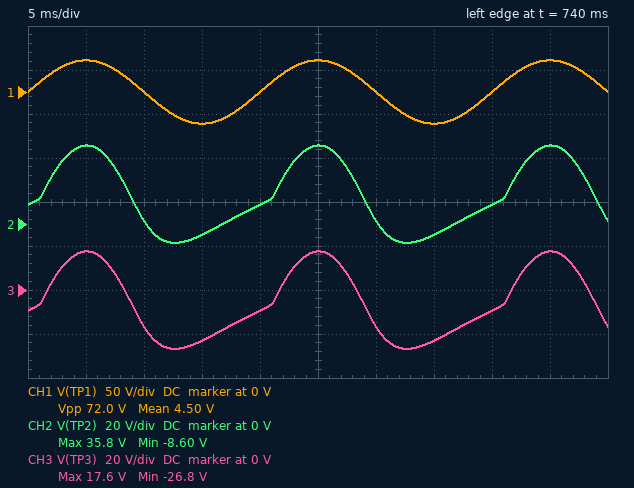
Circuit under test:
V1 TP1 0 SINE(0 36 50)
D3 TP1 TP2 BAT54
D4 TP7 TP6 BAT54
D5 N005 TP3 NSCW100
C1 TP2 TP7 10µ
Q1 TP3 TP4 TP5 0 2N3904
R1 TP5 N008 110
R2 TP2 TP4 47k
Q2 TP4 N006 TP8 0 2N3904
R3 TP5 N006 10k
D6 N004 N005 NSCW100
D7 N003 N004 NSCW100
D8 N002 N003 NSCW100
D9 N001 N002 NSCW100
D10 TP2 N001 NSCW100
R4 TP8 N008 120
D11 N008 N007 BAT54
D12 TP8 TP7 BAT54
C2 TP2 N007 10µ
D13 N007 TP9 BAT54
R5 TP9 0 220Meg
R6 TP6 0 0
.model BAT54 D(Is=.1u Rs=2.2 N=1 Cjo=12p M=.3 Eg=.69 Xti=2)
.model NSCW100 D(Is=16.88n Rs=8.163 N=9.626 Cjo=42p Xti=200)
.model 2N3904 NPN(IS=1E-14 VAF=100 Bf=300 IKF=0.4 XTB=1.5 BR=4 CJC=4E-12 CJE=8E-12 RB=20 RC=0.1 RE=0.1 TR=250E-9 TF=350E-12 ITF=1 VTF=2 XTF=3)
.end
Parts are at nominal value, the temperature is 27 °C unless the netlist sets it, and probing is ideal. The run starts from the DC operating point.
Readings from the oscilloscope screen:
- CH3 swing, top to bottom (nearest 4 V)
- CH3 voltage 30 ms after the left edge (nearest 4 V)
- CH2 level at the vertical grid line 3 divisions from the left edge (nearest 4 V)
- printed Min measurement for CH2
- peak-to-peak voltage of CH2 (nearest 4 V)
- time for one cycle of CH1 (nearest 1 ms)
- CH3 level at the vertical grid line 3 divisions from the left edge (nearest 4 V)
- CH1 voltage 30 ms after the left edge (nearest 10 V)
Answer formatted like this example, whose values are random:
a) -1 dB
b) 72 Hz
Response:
a) 44 V
b) -16 V
c) -4 V
d) -8.60 V
e) 44 V
f) 20 ms
g) -24 V
h) 0 V
